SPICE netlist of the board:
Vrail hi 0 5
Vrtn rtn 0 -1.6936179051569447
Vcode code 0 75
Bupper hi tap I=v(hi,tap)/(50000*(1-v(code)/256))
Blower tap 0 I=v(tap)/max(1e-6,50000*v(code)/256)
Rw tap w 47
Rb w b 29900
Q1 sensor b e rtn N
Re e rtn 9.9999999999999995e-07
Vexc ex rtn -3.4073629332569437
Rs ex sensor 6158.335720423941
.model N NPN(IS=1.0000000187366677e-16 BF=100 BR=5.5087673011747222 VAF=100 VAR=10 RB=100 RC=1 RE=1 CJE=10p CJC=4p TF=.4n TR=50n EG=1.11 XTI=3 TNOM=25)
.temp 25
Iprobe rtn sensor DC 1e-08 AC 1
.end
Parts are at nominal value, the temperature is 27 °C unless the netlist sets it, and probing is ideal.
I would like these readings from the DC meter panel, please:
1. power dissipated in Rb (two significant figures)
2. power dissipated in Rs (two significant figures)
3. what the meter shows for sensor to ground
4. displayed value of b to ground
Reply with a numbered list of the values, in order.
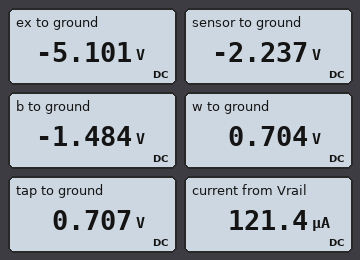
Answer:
1. 160 µW
2. 1.3 mW
3. -2.237 V
4. -1.484 V
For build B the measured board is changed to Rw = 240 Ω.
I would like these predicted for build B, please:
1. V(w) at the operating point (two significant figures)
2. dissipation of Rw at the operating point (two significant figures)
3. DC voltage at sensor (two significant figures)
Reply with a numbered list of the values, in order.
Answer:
1. 690 mV
2. 1.3 µW
3. -2.2 V
